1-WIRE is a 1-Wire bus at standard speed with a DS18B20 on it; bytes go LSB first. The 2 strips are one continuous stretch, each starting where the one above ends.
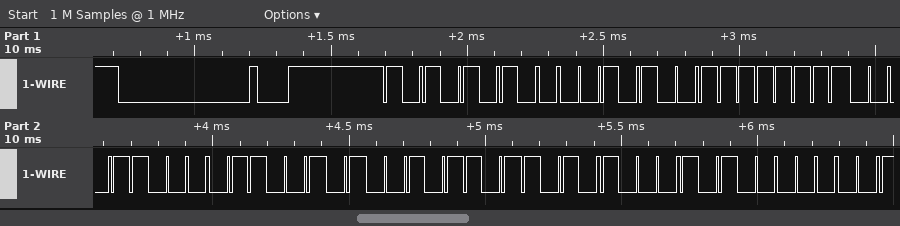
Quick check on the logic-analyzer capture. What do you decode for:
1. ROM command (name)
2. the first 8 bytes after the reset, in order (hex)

Match ROM
55 28 FF 18 A6 B4 15 05
